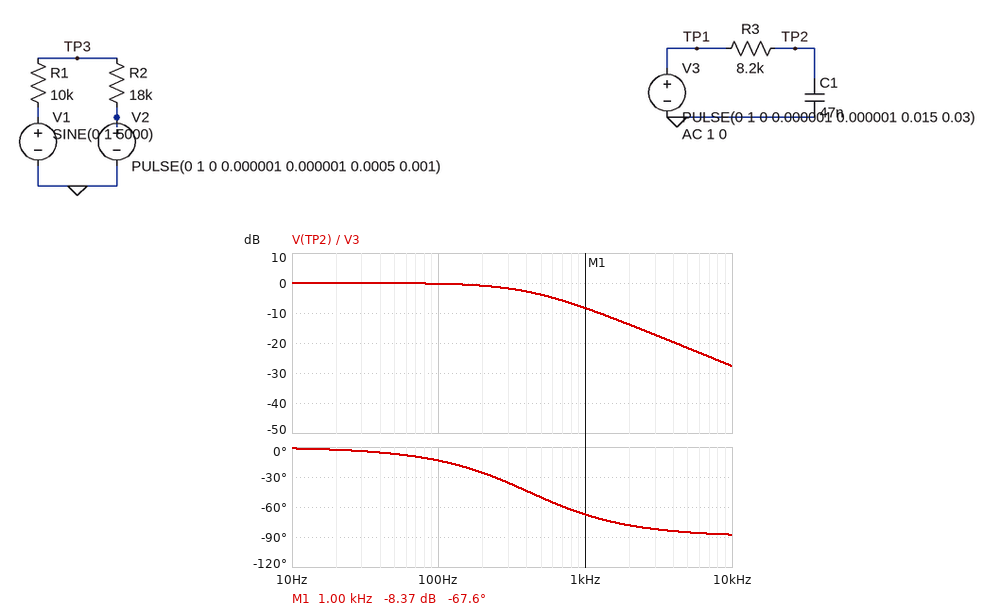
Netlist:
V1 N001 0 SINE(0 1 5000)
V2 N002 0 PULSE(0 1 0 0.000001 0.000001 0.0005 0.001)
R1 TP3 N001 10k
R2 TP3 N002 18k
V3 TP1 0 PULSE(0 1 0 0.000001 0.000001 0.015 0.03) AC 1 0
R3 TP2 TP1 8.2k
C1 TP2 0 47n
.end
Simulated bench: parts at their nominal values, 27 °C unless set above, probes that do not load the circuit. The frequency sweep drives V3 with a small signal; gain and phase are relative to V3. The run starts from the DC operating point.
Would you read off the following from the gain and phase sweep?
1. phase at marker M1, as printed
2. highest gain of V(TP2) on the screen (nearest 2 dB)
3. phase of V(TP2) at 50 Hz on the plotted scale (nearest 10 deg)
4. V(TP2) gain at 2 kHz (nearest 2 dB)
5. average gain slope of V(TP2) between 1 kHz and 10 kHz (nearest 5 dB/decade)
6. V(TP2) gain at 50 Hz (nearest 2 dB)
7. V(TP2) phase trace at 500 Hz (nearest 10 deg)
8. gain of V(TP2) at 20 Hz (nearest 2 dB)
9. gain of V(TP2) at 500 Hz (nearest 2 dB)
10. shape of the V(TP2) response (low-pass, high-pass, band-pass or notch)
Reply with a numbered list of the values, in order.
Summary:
1. -67.6 deg
2. 0 dB
3. -10 deg
4. -14 dB
5. -20 dB/decade
6. 0 dB
7. -50 deg
8. 0 dB
9. -4 dB
10. low-pass
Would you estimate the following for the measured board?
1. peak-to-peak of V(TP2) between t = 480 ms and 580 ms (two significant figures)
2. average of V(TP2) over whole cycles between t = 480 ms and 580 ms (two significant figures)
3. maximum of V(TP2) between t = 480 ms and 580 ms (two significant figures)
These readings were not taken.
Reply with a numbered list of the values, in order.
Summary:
1. 1.0 V
2. 500 mV
3. 1.0 V
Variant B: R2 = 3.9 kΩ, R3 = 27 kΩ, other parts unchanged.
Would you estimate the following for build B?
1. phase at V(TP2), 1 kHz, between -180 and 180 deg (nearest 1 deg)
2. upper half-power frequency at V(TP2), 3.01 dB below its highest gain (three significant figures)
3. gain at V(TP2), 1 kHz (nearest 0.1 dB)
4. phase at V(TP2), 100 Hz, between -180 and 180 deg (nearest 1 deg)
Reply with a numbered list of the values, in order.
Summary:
1. -83 deg
2. 125 Hz
3. -18.1 dB
4. -39 deg
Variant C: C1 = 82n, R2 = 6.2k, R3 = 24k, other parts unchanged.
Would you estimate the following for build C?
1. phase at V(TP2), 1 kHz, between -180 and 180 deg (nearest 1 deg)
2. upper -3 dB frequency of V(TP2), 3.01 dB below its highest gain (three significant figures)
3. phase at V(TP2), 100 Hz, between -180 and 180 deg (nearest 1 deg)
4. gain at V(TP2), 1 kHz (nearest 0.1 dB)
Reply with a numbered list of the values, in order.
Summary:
1. -85 deg
2. 80.9 Hz
3. -51 deg
4. -21.9 dB
